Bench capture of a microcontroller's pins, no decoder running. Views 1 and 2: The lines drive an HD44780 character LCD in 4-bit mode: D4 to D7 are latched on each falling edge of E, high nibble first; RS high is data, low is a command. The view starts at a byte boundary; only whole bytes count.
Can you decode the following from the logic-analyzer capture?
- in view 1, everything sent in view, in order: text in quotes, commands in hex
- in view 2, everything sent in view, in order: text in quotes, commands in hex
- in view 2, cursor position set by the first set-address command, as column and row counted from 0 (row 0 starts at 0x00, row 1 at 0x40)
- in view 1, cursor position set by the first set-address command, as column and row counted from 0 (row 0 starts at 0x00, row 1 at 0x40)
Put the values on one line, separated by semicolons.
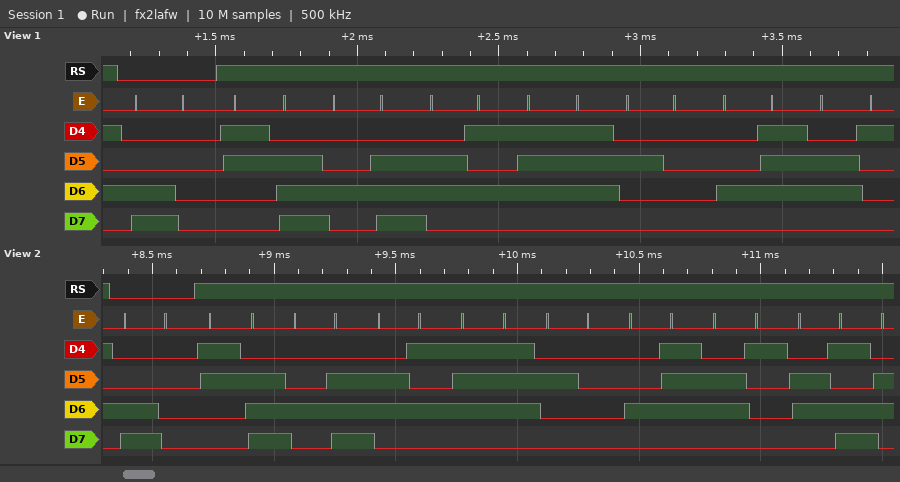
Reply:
0xC0 ">New Ga"; 0xC0 ">New Gam"; column 0, row 1; column 0, row 1
